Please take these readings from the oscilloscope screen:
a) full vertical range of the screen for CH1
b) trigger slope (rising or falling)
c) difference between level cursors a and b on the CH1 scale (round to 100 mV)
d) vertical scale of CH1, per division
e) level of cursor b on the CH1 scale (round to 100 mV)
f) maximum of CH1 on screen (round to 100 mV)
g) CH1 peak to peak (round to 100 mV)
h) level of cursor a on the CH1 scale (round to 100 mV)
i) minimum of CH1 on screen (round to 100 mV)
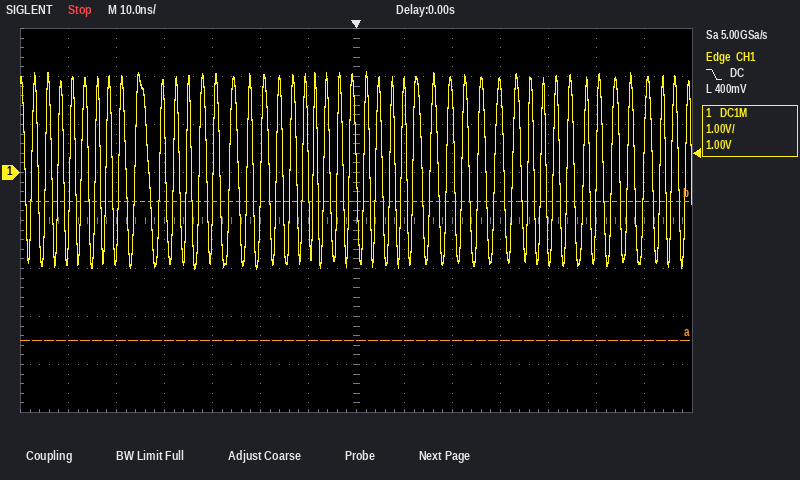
8 V
falling
2.9 V
1 V
-600 mV
2.1 V
4.1 V
-3.5 V
-2.0 V
